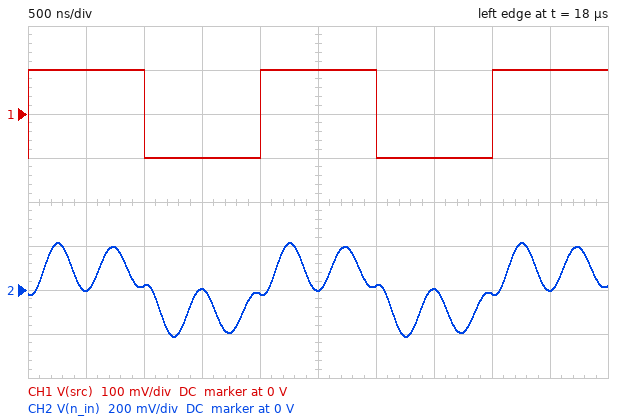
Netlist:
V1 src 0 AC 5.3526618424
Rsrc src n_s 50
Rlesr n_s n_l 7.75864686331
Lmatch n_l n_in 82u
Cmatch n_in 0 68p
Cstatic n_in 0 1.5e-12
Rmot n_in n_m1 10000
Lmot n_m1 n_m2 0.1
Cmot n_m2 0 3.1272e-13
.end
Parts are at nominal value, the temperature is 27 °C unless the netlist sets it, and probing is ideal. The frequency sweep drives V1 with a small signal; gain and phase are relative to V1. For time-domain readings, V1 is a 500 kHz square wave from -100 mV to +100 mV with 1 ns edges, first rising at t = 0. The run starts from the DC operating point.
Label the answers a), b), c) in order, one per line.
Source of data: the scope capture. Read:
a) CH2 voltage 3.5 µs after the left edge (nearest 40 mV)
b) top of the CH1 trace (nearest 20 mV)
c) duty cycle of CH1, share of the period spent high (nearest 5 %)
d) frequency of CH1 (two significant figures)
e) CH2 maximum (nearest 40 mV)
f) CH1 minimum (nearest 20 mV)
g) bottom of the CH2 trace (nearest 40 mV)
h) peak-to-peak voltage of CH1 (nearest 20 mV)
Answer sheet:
a) 0 V
b) 100 mV
c) 50 %
d) 500 kHz
e) 200 mV
f) -100 mV
g) -200 mV
h) 200 mV
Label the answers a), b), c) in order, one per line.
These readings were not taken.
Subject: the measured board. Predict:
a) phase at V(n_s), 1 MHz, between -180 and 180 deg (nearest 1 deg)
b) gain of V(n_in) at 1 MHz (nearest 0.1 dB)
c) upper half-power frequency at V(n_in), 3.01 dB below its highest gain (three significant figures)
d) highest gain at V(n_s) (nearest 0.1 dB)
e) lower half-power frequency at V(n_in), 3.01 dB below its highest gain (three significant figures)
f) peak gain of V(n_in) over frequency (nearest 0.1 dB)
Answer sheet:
a) -2 deg
b) 2.2 dB
c) 2.16 MHz
d) 0 dB
e) 2.05 MHz
f) 25.5 dB
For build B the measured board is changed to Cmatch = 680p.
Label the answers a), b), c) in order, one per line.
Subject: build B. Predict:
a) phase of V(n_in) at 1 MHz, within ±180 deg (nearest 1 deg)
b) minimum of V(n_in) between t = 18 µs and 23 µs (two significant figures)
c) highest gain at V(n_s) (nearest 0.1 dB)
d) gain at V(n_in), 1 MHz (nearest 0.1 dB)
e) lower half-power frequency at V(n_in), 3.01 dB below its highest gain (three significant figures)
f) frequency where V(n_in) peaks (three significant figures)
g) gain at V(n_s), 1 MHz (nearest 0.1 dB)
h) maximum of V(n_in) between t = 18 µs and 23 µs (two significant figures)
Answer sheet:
a) -168 deg
b) -280 mV
c) 0 dB
d) -1.8 dB
e) 609 kHz
f) 668 kHz
g) -0.2 dB
h) 280 mV
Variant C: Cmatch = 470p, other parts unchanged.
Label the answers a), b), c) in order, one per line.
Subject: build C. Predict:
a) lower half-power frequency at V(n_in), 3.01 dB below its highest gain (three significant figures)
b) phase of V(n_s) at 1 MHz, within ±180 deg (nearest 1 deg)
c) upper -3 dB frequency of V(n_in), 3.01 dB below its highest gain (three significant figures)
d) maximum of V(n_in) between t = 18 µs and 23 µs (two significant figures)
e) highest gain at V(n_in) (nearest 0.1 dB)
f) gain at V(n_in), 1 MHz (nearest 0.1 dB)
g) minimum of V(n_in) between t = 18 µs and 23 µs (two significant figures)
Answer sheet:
a) 746 kHz
b) 16 deg
c) 857 kHz
d) 220 mV
e) 17.2 dB
f) 5.2 dB
g) -220 mV
